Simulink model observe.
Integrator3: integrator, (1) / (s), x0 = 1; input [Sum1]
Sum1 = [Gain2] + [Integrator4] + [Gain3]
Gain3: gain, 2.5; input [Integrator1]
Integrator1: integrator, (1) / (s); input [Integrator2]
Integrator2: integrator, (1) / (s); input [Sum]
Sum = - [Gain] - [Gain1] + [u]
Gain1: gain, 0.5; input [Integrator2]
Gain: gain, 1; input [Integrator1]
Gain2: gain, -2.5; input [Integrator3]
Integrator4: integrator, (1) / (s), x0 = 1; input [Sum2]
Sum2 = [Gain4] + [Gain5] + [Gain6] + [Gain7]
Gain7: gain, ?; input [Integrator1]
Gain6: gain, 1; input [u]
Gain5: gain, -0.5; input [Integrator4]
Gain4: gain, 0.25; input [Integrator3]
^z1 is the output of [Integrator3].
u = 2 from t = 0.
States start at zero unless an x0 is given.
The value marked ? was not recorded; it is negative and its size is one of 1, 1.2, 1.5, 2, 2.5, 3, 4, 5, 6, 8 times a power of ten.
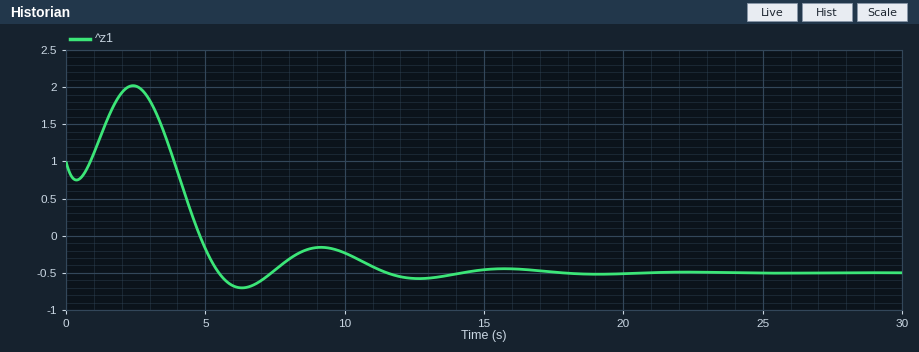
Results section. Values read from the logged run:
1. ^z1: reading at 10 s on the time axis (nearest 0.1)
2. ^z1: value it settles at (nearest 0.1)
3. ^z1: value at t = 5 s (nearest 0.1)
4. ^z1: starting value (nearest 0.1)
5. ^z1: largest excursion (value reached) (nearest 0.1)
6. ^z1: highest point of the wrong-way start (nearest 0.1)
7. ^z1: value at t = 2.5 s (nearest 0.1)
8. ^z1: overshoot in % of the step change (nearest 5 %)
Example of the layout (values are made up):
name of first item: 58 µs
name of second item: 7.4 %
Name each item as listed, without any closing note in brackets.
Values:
^z1: reading at 10 s on the time axis: -0.2
^z1: value it settles at: -0.5
^z1: value at t = 5 s: -0.2
^z1: starting value: 1.0
^z1: largest excursion (value reached): -0.7
^z1: highest point of the wrong-way start: 2.0
^z1: value at t = 2.5 s: 2.0
^z1: overshoot in % of the step change: 15 %
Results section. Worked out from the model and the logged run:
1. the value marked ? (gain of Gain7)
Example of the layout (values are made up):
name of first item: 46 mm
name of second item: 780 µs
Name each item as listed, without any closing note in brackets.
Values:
the value marked ?: -2.5
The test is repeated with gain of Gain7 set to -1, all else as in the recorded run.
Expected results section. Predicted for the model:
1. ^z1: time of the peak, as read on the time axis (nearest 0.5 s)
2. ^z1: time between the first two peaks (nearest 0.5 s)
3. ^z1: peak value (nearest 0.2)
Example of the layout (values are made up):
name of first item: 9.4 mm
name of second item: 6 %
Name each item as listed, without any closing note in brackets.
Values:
^z1: time of the peak, as read on the time axis: 3.5 s
^z1: time between the first two peaks: 6.5 s
^z1: peak value: 3.4
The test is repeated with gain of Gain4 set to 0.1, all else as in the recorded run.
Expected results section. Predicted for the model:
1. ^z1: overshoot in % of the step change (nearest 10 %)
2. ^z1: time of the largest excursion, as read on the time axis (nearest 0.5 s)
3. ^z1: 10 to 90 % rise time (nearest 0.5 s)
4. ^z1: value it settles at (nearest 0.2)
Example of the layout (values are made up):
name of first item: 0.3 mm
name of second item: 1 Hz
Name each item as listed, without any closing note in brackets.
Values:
^z1: overshoot in % of the step change: 20 %
^z1: time of the largest excursion, as read on the time axis: 6.0 s
^z1: 10 to 90 % rise time: 5.0 s
^z1: value it settles at: -0.4
